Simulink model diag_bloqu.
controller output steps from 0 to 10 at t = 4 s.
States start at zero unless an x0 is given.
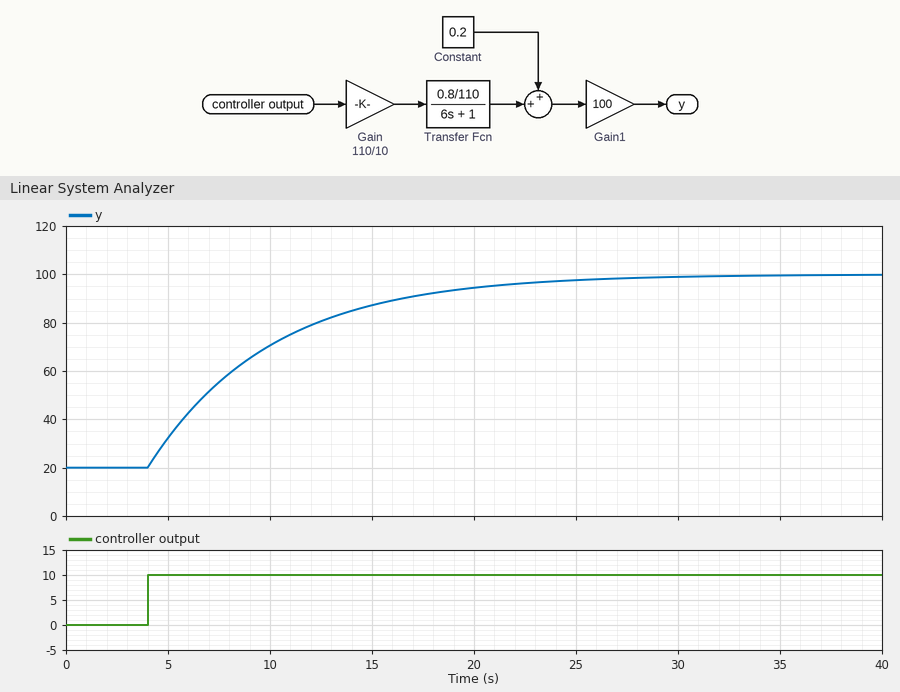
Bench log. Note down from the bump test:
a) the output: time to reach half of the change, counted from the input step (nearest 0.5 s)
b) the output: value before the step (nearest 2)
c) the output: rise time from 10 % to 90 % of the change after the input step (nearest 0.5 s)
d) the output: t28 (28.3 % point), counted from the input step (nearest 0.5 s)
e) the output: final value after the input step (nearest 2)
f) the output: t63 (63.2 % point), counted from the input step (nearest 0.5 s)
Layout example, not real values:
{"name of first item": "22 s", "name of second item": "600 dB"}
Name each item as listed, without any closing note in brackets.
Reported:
{"the output: time to reach half of the change, counted from the input step": "4.0 s", "the output: value before the step": "20", "the output: rise time from 10 % to 90 % of the change after the input step": "13.0 s", "the output: t28 (28.3 % point), counted from the input step": "2.0 s", "the output: final value after the input step": "100", "the output: t63 (63.2 % point), counted from the input step": "6.0 s"}
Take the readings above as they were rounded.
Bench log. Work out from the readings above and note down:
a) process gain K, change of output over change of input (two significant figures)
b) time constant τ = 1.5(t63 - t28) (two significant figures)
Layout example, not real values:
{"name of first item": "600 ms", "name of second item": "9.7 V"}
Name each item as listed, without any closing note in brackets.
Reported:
{"process gain K, change of output over change of input": "8.0", "time constant τ = 1.5(t63 - t28)": "6.0 s"}
